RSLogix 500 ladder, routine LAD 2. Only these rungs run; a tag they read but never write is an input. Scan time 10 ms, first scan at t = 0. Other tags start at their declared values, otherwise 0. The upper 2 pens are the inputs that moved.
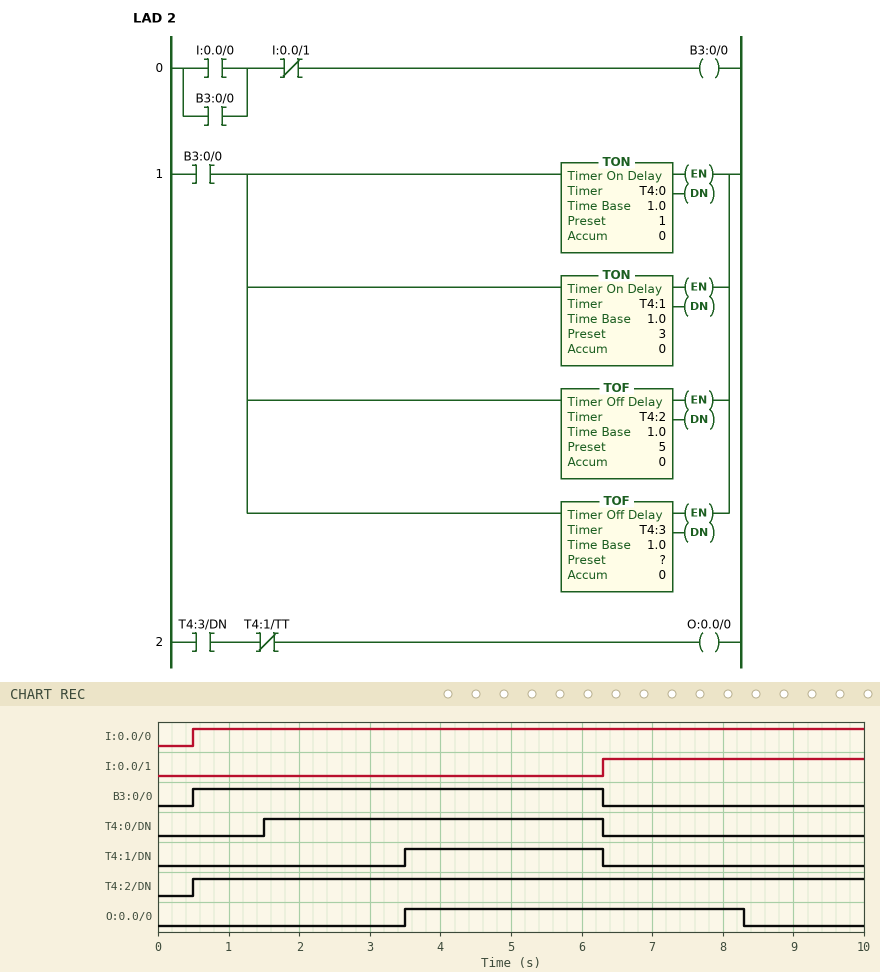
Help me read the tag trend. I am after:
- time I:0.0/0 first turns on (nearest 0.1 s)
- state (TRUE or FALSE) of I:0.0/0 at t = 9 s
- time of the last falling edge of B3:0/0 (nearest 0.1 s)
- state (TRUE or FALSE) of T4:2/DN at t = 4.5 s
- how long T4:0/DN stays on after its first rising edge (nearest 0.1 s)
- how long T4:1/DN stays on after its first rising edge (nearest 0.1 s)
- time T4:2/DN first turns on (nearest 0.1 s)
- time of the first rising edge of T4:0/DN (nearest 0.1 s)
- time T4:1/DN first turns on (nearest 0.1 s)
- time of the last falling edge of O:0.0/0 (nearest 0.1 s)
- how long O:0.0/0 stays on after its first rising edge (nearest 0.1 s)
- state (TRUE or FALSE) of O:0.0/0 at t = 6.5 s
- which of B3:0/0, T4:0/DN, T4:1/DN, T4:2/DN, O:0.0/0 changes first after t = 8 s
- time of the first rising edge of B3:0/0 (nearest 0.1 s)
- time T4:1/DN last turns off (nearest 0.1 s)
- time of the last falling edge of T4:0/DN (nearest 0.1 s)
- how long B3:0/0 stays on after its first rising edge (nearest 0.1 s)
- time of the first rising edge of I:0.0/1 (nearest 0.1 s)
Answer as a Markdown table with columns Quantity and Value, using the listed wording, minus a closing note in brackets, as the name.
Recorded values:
| Quantity | Value |
|---|---|
| time I:0.0/0 first turns on | 0.5 s |
| state (TRUE or FALSE) of I:0.0/0 at t = 9 s | TRUE |
| time of the last falling edge of B3:0/0 | 6.3 s |
| state (TRUE or FALSE) of T4:2/DN at t = 4.5 s | TRUE |
| how long T4:0/DN stays on after its first rising edge | 4.8 s |
| how long T4:1/DN stays on after its first rising edge | 2.8 s |
| time T4:2/DN first turns on | 0.5 s |
| time of the first rising edge of T4:0/DN | 1.5 s |
| time T4:1/DN first turns on | 3.5 s |
| time of the last falling edge of O:0.0/0 | 8.3 s |
| how long O:0.0/0 stays on after its first rising edge | 4.8 s |
| state (TRUE or FALSE) of O:0.0/0 at t = 6.5 s | TRUE |
| which of B3:0/0, T4:0/DN, T4:1/DN, T4:2/DN, O:0.0/0 changes first after t = 8 s | O:0.0/0 |
| time of the first rising edge of B3:0/0 | 0.5 s |
| time T4:1/DN last turns off | 6.3 s |
| time of the last falling edge of T4:0/DN | 6.3 s |
| how long B3:0/0 stays on after its first rising edge | 5.8 s |
| time of the first rising edge of I:0.0/1 | 6.3 s |
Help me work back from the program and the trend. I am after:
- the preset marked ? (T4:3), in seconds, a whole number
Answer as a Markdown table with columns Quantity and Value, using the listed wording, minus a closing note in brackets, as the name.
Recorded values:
| Quantity | Value |
|---|---|
| the preset marked ? (T4:3), in seconds, a whole number | 2 s |
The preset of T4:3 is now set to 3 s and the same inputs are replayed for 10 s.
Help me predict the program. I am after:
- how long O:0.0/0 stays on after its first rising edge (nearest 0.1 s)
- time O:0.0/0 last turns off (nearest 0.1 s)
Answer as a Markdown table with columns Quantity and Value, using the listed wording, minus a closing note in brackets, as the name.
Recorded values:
| Quantity | Value |
|---|---|
| how long O:0.0/0 stays on after its first rising edge | 5.8 s |
| time O:0.0/0 last turns off | 9.3 s |
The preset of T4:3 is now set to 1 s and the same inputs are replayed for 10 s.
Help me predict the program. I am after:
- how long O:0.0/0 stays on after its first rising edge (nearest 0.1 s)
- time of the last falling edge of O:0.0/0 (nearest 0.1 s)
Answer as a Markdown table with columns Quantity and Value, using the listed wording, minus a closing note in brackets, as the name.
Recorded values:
| Quantity | Value |
|---|---|
| how long O:0.0/0 stays on after its first rising edge | 3.8 s |
| time of the last falling edge of O:0.0/0 | 7.3 s |
